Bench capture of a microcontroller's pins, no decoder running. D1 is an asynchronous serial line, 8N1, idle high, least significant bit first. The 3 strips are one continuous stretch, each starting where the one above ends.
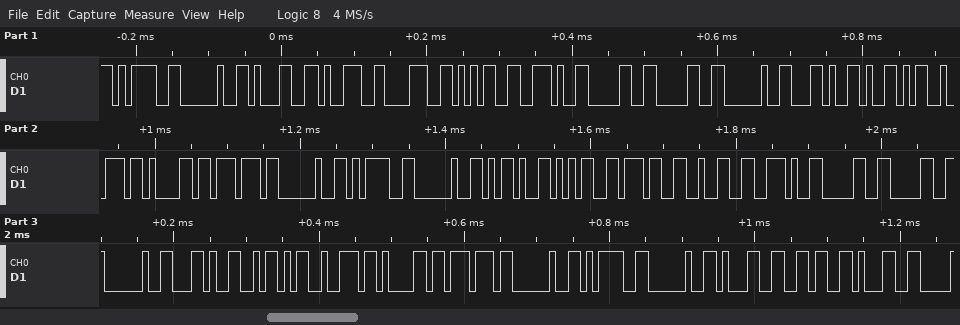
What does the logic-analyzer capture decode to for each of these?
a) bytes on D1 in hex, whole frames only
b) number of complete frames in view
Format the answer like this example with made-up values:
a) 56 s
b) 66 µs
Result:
a) 3D 20 31 39 38 35 2E 30 30 20 2C 59 72 61 77 20 3D 20 2D 35 37 32 2E 30 30 20 2C 5A 72 61 77 20 3D 20 31 36 31
b) 37
